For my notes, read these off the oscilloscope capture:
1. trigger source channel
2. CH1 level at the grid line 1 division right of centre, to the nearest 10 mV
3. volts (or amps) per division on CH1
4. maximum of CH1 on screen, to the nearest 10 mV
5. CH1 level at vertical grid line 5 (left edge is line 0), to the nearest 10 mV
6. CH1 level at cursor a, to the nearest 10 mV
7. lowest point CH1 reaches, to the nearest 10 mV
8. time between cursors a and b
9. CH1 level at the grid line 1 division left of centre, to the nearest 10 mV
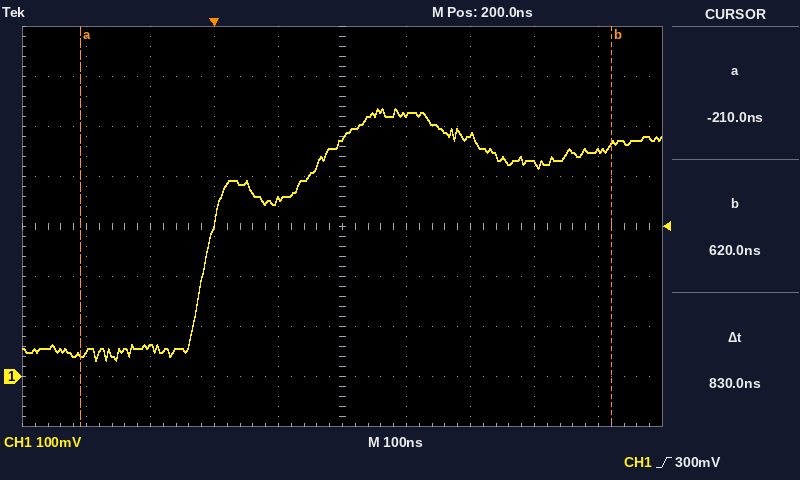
CH1
520 mV
100 mV
540 mV
480 mV
40 mV
30 mV
830 ns
350 mV
